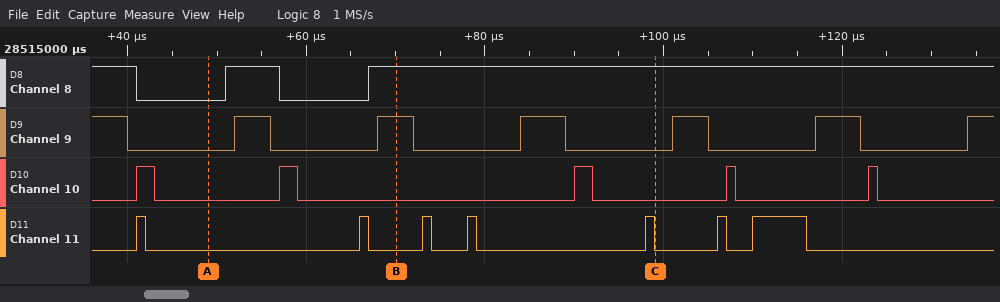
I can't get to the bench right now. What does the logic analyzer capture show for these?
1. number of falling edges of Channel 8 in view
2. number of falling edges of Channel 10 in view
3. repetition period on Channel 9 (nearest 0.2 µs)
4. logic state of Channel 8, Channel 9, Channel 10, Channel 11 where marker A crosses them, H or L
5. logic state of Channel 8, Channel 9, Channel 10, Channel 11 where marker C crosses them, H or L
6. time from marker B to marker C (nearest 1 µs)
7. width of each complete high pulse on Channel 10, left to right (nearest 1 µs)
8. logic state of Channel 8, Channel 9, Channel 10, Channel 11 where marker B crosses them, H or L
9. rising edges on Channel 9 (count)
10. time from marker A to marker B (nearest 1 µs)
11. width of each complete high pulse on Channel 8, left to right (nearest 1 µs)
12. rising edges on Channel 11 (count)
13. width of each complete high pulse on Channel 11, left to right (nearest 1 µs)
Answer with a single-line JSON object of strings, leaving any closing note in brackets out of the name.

{"number of falling edges of Channel 8 in view": "2", "number of falling edges of Channel 10 in view": "5", "repetition period on Channel 9": "16.4 µs", "logic state of Channel 8, Channel 9, Channel 10, Channel 11 where marker A crosses them, H or L": "Channel 8=L, Channel 9=L, Channel 10=L, Channel 11=L", "logic state of Channel 8, Channel 9, Channel 10, Channel 11 where marker C crosses them, H or L": "Channel 8=H, Channel 9=L, Channel 10=L, Channel 11=L", "time from marker B to marker C": "29 µs", "width of each complete high pulse on Channel 10, left to right": "2 µs, 2 µs, 2 µs, 1 µs, 1 µs", "logic state of Channel 8, Channel 9, Channel 10, Channel 11 where marker B crosses them, H or L": "Channel 8=H, Channel 9=H, Channel 10=L, Channel 11=L", "rising edges on Channel 9": "6", "time from marker A to marker B": "21 µs", "width of each complete high pulse on Channel 8, left to right": "6 µs", "rising edges on Channel 11": "7", "width of each complete high pulse on Channel 11, left to right": "1 µs, 1 µs, 1 µs, 1 µs, 1 µs, 1 µs, 6 µs"}
